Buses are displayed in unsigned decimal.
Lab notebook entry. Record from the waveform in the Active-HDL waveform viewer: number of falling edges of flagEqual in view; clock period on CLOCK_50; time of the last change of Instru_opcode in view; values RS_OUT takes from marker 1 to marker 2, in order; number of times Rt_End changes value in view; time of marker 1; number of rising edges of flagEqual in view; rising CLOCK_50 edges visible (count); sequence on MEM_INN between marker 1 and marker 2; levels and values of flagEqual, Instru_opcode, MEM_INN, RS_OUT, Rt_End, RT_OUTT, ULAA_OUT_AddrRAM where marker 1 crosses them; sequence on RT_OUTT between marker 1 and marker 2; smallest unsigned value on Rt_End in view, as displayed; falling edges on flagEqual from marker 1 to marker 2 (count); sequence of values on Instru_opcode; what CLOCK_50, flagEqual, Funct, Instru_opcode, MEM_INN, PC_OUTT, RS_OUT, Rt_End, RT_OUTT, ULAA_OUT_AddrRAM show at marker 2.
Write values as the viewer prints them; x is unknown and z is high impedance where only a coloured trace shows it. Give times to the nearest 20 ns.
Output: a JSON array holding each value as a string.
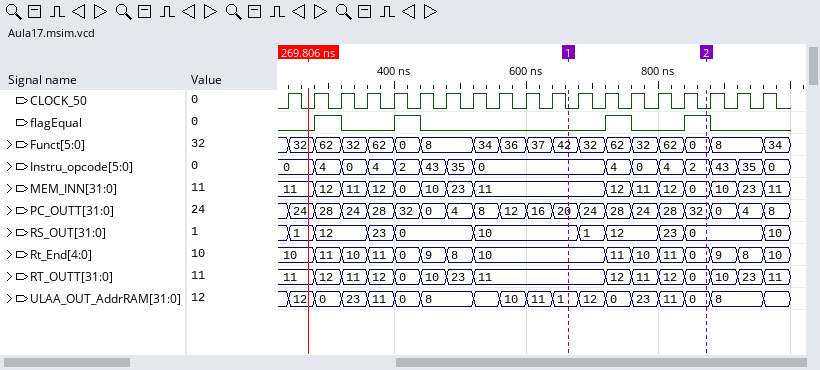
["4", "40 ns", "960 ns", "10, 1, 12, 23, 0", "14", "660 ns", "4", "19", "11, 12, 11, 12, 0", "flagEqual=0, Instru_opcode=0, MEM_INN=11, RS_OUT=10, Rt_End=10, RT_OUTT=11, ULAA_OUT_AddrRAM=1", "11, 12, 11, 12, 0", "0", "1", "0, 4, 0, 4, 2, 43, 35, 0, 4, 0, 4, 2, 43, 35, 0", "CLOCK_50=0, flagEqual=1, Funct=0, Instru_opcode=2, MEM_INN=0, PC_OUTT=32, RS_OUT=0, Rt_End=0, RT_OUTT=0, ULAA_OUT_AddrRAM=0"]
